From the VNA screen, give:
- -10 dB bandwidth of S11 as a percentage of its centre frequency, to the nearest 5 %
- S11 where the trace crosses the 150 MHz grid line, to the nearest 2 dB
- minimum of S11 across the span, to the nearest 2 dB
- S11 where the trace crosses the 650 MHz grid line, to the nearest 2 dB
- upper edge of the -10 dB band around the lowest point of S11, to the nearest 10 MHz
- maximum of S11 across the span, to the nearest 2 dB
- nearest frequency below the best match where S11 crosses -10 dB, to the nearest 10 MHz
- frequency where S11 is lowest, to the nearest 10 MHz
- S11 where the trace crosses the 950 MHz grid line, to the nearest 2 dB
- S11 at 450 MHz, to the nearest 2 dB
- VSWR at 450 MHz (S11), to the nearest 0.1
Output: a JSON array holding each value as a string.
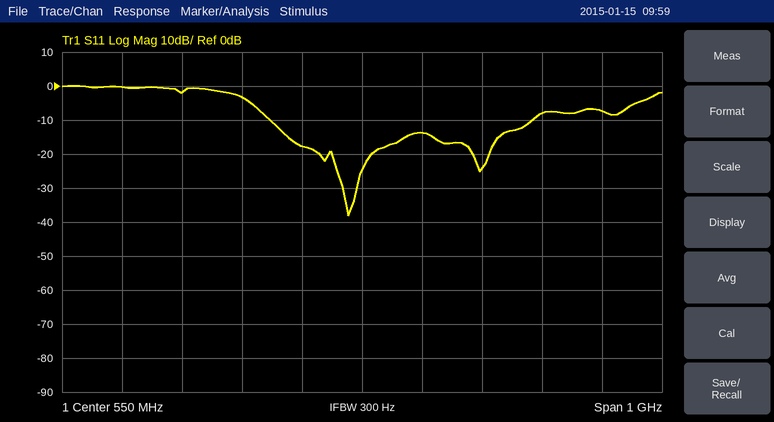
["70 %", "0 dB", "-38 dB", "-14 dB", "830 MHz", "0 dB", "400 MHz", "530 MHz", "-8 dB", "-18 dB", "1.3"]
